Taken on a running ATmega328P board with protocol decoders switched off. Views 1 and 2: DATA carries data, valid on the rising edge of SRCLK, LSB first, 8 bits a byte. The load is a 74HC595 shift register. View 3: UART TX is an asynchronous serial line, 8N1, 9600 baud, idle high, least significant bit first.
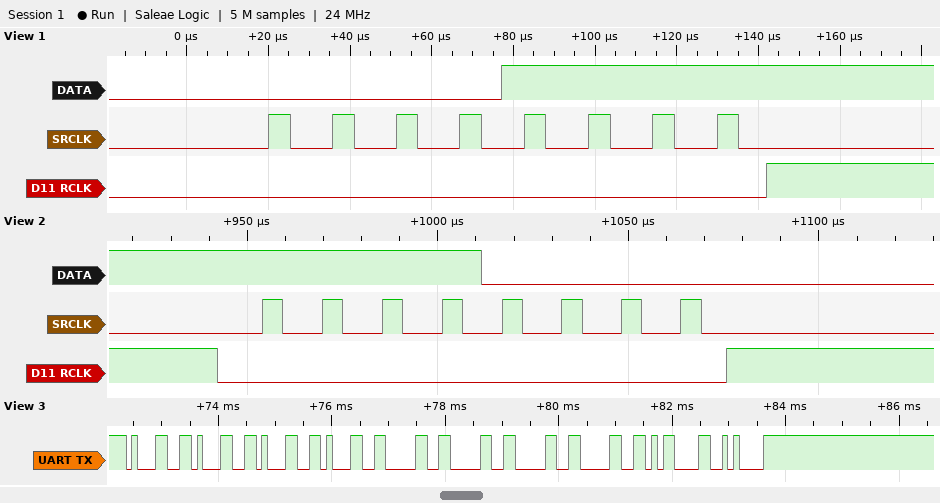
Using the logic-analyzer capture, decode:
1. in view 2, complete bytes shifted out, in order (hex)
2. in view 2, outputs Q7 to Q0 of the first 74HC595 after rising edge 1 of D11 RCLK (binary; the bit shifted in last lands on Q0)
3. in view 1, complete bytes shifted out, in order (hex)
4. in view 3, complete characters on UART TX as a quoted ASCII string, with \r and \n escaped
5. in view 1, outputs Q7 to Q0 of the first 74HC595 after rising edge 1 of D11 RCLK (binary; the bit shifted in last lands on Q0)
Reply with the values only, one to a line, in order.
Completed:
0F
11110000
F0
"11110000\r\n"
00001111
